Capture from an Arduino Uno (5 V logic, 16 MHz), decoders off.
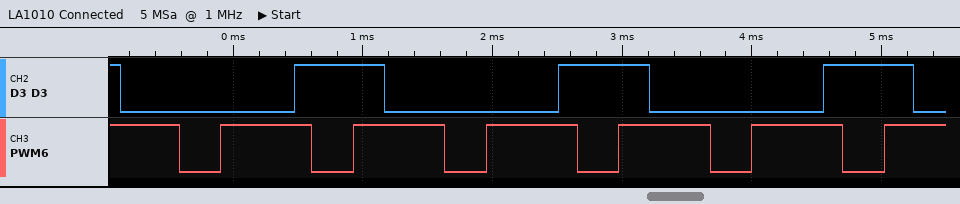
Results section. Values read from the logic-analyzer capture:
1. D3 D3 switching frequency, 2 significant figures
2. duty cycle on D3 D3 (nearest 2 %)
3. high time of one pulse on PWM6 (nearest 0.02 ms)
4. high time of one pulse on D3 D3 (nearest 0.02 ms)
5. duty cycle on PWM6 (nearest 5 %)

490 Hz
34 %
0.70 ms
0.70 ms
70 %
